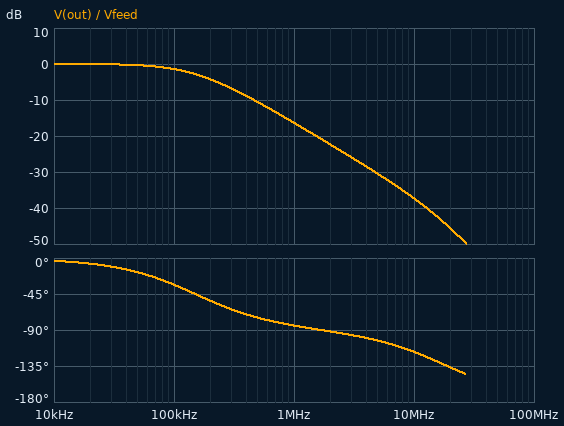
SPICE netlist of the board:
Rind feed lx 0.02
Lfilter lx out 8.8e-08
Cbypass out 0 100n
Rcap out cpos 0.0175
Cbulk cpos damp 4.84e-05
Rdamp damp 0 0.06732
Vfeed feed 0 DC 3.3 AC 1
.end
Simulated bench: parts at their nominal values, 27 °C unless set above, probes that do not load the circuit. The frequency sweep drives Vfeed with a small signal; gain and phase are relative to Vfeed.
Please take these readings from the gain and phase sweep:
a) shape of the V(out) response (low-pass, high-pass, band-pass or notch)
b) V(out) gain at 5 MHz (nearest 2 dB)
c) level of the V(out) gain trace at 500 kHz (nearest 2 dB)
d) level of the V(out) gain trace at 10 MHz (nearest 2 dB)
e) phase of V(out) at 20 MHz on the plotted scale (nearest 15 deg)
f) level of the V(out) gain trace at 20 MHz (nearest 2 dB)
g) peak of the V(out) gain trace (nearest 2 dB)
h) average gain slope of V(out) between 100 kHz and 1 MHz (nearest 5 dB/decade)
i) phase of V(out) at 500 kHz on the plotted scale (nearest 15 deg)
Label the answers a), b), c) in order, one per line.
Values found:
a) low-pass
b) -30 dB
c) -10 dB
d) -38 dB
e) -135 deg
f) -46 dB
g) 0 dB
h) -15 dB/decade
i) -75 deg
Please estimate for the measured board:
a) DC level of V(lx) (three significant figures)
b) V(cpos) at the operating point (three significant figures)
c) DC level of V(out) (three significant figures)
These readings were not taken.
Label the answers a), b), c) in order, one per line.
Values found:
a) 3.30 V
b) 3.30 V
c) 3.30 V
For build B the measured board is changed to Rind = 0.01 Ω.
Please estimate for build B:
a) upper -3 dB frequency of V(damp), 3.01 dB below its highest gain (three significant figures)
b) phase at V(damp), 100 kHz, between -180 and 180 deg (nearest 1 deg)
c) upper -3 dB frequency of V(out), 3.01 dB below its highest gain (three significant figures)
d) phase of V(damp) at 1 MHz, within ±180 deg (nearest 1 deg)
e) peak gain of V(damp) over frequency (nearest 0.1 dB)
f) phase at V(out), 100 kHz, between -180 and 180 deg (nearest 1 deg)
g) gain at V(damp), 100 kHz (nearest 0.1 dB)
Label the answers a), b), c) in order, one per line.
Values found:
a) 202 kHz
b) -13 deg
c) 162 kHz
d) -83 deg
e) -3.0 dB
f) -35 deg
g) -3.2 dB
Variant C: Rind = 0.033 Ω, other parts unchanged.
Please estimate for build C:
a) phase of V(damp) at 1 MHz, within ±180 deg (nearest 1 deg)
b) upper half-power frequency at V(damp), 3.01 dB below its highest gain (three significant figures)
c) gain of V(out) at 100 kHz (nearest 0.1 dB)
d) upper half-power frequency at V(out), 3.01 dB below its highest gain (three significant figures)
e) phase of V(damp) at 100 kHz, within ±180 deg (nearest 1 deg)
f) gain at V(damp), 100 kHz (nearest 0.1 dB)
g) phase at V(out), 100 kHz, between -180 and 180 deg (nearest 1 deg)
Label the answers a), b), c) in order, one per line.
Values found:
a) -81 deg
b) 239 kHz
c) -2.4 dB
d) 126 kHz
e) -11 deg
f) -5.0 dB
g) -32 deg
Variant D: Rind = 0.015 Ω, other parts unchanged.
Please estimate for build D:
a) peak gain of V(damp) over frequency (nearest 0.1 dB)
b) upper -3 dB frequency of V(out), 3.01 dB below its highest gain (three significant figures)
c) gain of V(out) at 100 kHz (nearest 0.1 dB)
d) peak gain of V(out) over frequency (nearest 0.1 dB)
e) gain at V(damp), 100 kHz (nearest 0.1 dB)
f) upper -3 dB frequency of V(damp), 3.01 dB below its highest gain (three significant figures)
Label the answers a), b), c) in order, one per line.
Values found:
a) -3.4 dB
b) 163 kHz
c) -1.0 dB
d) 0.1 dB
e) -3.6 dB
f) 210 kHz
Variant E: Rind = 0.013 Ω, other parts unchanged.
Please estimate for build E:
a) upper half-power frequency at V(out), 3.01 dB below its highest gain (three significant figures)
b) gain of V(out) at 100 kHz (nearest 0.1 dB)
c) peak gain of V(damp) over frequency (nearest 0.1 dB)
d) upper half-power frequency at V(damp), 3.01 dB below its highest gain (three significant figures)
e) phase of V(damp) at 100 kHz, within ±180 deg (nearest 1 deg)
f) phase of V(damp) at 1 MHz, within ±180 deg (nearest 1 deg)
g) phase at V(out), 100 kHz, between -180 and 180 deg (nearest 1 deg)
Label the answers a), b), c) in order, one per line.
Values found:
a) 163 kHz
b) -0.8 dB
c) -3.2 dB
d) 207 kHz
e) -13 deg
f) -83 deg
g) -34 deg
